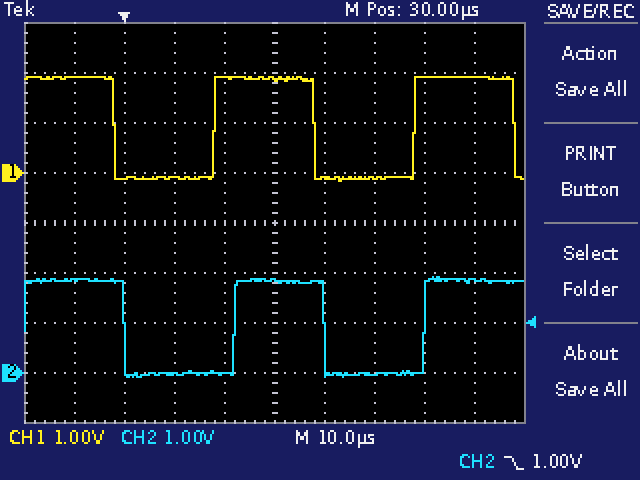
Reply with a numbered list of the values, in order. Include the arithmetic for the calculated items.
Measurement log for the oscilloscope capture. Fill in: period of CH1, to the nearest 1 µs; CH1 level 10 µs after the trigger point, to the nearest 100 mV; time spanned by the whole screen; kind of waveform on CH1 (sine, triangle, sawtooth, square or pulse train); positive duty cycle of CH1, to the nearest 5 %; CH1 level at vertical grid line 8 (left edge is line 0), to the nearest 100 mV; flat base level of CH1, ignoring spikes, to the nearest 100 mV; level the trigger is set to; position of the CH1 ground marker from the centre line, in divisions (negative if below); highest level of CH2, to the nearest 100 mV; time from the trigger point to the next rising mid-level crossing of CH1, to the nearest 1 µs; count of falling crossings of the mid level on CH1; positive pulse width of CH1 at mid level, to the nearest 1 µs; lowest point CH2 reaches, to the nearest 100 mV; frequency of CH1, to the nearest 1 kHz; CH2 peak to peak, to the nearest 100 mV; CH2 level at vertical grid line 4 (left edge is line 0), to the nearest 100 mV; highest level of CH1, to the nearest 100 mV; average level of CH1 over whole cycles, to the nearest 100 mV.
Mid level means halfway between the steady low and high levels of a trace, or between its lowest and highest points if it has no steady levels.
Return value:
1. 40 µs
2. -100 mV
3. 100 µs
4. square
5. 20 µs / 40 µs ≈ 50 %
6. 1.9 V
7. -100 mV
8. 1.00 V
9. +1.0 div
10. 1.9 V
11. 18 µs
12. 3
13. 20 µs
14. -100 mV
15. 1 / 40 µs ≈ 25 kHz
16. 1.9 V − (-100 mV) = 2.0 V
17. 0.0 V
18. 1.9 V
19. -100 mV + 0.5 × (1.9 V − (-100 mV)) ≈ 900 mV
